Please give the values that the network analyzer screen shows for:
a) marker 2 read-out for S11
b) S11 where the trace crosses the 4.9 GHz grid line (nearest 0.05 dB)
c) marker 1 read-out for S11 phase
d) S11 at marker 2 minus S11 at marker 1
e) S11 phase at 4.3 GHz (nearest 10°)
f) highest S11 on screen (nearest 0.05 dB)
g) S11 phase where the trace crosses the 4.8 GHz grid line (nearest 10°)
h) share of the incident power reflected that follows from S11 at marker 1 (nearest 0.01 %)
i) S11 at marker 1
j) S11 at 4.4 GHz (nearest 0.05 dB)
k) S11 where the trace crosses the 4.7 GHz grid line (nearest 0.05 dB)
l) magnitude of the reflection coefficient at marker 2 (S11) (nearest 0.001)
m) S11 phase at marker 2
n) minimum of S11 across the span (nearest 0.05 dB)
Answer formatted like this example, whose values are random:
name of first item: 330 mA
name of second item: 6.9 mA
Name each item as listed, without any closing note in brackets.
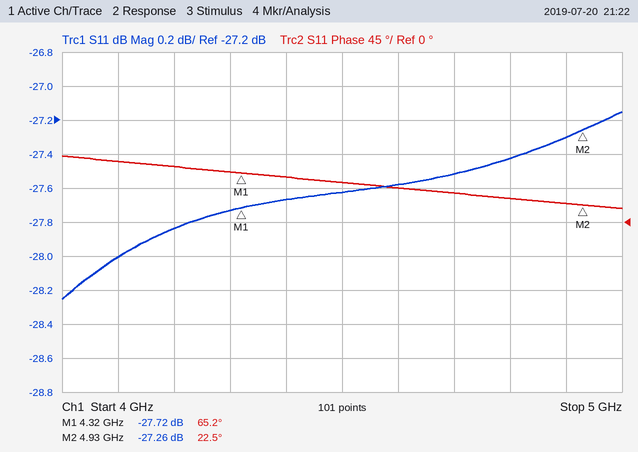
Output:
marker 2 read-out for S11: -27.26 dB
S11 where the trace crosses the 4.9 GHz grid line: -27.30 dB
marker 1 read-out for S11 phase: 65.2°
S11 at marker 2 minus S11 at marker 1: 0.46 dB
S11 phase at 4.3 GHz: 70°
highest S11 on screen: -27.15 dB
S11 phase where the trace crosses the 4.8 GHz grid line: 30°
share of the incident power reflected that follows from S11 at marker 1: 0.17 %
S11 at marker 1: -27.72 dB
S11 at 4.4 GHz: -27.65 dB
S11 where the trace crosses the 4.7 GHz grid line: -27.50 dB
magnitude of the reflection coefficient at marker 2 (S11): 0.043
S11 phase at marker 2: 22.5°
minimum of S11 across the span: -28.25 dB
